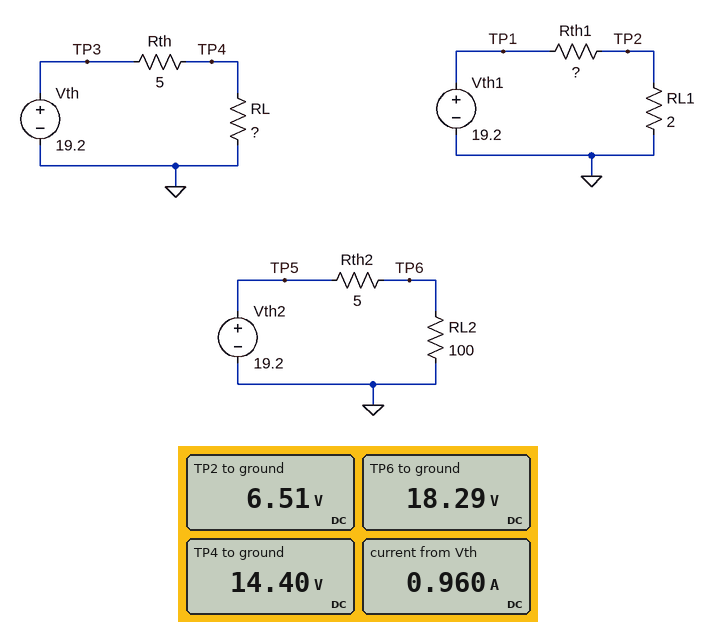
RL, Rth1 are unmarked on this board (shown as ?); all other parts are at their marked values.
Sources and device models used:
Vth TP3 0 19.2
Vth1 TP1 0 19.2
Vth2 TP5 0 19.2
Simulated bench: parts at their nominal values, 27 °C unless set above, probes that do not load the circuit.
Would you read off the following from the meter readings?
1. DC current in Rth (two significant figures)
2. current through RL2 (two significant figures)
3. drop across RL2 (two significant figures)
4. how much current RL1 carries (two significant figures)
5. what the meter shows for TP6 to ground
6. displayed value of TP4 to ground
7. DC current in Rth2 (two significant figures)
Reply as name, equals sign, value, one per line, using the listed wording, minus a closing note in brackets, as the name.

DC current in Rth = 960 mA
current through RL2 = 180 mA
drop across RL2 = 18 V
how much current RL1 carries = 3.3 A
what the meter shows for TP6 to ground = 18.29 V
displayed value of TP4 to ground = 14.40 V
DC current in Rth2 = 180 mA
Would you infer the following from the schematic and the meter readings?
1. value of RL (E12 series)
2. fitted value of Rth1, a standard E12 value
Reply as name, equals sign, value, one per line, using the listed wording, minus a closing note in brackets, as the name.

value of RL = 15 Ω
fitted value of Rth1, a standard E12 value = 3.9 Ω
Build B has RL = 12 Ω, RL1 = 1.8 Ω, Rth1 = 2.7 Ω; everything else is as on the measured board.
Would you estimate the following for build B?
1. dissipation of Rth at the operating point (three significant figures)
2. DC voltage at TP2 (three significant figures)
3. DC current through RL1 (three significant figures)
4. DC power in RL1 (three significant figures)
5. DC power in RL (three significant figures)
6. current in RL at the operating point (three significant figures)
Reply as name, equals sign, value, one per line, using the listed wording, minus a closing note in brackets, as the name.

dissipation of Rth at the operating point = 6.38 W
DC voltage at TP2 = 7.68 V
DC current through RL1 = 4.27 A
DC power in RL1 = 32.8 W
DC power in RL = 15.3 W
current in RL at the operating point = 1.13 A
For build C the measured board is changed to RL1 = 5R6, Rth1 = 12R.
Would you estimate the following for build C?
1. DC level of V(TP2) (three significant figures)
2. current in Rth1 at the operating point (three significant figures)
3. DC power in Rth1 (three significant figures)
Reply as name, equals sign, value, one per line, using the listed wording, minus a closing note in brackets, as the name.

DC level of V(TP2) = 6.11 V
current in Rth1 at the operating point = 1.09 A
DC power in Rth1 = 14.3 W
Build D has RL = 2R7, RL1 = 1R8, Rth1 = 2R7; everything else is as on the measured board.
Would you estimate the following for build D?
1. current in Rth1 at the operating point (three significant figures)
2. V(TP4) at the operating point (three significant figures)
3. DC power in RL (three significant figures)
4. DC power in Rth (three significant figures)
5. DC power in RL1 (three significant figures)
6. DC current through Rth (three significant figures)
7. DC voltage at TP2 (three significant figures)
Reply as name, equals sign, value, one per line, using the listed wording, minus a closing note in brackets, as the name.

current in Rth1 at the operating point = 4.27 A
V(TP4) at the operating point = 6.73 V
DC power in RL = 16.8 W
DC power in Rth = 31.1 W
DC power in RL1 = 32.8 W
DC current through Rth = 2.49 A
DC voltage at TP2 = 7.68 V
